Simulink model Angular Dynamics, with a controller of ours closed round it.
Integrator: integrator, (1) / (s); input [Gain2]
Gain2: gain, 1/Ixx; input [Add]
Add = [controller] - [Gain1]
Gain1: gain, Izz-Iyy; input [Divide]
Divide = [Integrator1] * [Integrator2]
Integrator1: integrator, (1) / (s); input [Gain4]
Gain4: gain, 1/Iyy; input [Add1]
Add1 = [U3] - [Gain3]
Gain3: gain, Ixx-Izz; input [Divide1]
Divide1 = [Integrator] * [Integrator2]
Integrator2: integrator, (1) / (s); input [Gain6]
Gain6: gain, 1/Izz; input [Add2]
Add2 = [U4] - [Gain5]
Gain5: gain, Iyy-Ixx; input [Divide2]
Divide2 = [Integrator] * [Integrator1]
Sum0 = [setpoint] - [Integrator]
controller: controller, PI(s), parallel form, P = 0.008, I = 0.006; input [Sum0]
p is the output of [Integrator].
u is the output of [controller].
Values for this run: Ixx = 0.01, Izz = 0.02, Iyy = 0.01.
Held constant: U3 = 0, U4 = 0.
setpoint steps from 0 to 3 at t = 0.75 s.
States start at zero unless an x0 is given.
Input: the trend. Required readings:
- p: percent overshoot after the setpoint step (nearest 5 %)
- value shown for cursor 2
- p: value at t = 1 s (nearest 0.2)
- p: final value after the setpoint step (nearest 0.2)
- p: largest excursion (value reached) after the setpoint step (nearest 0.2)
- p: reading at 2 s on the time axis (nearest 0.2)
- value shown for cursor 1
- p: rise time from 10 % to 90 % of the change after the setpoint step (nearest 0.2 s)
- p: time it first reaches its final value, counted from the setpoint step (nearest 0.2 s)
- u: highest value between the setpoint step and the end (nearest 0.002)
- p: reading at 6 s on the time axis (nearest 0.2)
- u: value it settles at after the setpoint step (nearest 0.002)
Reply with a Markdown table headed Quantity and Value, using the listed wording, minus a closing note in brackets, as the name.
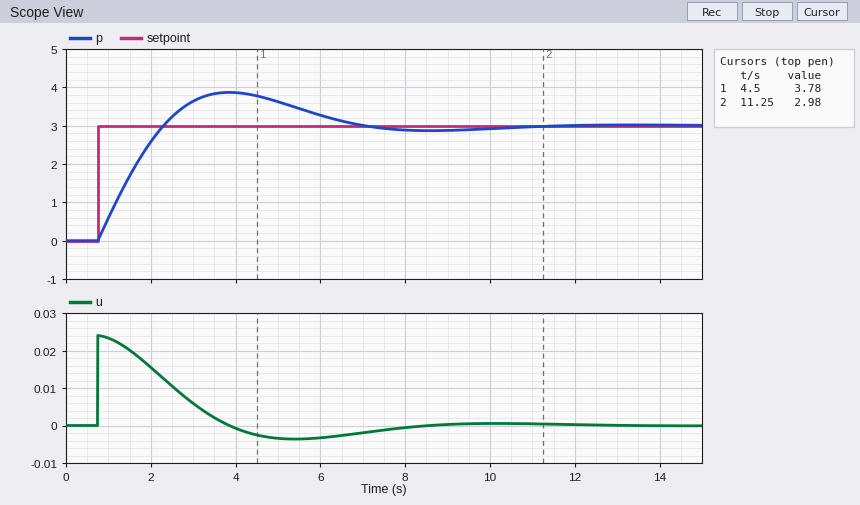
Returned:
| Quantity | Value |
|---|---|
| p: percent overshoot after the setpoint step | 30 % |
| value shown for cursor 2 | 2.98 |
| p: value at t = 1 s | 0.6 |
| p: final value after the setpoint step | 3.0 |
| p: largest excursion (value reached) after the setpoint step | 3.8 |
| p: reading at 2 s on the time axis | 2.6 |
| value shown for cursor 1 | 3.78 |
| p: rise time from 10 % to 90 % of the change after the setpoint step | 1.2 s |
| p: time it first reaches its final value, counted from the setpoint step | 1.6 s |
| u: highest value between the setpoint step and the end | 0.024 |
| p: reading at 6 s on the time axis | 3.2 |
| u: value it settles at after the setpoint step | 0.000 |
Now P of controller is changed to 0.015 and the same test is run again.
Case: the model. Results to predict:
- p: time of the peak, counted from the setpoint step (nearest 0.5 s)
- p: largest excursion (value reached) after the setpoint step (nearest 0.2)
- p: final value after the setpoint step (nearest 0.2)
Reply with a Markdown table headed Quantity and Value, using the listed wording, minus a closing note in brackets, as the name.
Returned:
| Quantity | Value |
|---|---|
| p: time of the peak, counted from the setpoint step | 2.5 s |
| p: largest excursion (value reached) after the setpoint step | 3.4 |
| p: final value after the setpoint step | 3.0 |
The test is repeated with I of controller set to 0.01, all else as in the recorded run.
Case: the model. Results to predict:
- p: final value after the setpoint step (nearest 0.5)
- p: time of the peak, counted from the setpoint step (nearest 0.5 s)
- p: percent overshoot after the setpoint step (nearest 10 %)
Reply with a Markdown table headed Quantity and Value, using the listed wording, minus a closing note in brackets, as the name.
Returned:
| Quantity | Value |
|---|---|
| p: final value after the setpoint step | 3.0 |
| p: time of the peak, counted from the setpoint step | 2.5 s |
| p: percent overshoot after the setpoint step | 40 % |
